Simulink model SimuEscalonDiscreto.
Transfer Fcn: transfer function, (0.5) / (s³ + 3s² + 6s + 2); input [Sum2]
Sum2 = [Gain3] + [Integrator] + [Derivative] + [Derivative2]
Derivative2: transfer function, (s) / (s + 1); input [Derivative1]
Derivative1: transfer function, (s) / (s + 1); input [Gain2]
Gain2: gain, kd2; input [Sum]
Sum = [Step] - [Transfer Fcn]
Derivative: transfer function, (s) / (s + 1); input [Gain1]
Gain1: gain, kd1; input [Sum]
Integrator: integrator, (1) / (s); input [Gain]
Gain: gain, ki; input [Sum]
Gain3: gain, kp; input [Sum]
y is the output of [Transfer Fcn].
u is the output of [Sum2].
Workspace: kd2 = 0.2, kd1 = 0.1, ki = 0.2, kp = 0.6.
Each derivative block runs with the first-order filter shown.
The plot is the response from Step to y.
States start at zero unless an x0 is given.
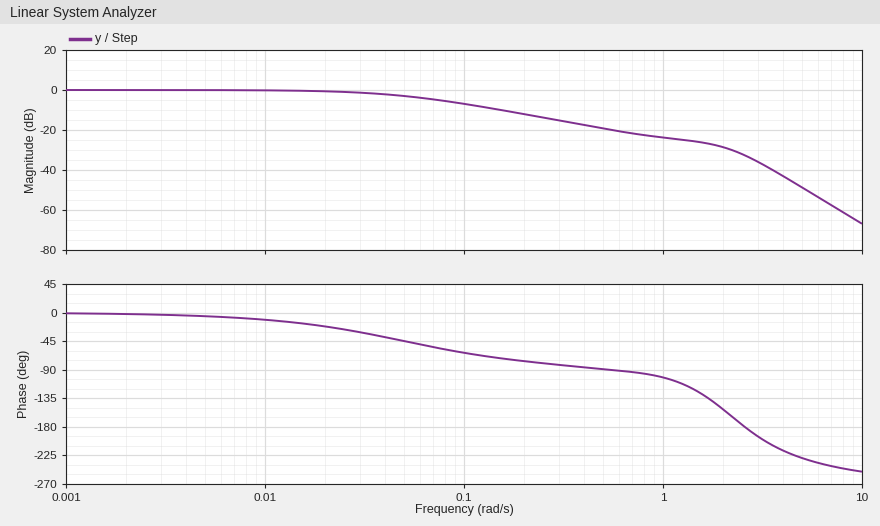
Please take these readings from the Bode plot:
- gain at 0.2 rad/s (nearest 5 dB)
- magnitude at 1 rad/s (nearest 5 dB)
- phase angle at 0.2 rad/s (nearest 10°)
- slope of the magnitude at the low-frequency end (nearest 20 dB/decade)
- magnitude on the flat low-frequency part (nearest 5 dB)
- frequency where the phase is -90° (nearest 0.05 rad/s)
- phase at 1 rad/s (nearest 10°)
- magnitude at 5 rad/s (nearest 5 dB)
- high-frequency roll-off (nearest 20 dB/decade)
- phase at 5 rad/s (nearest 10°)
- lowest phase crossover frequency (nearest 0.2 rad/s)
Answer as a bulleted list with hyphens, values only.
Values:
- -10 dB
- -25 dB
- -80°
- 0 dB/decade
- 0 dB
- 0.55 rad/s
- -100°
- -50 dB
- -60 dB/decade
- -230°
- 2.6 rad/s
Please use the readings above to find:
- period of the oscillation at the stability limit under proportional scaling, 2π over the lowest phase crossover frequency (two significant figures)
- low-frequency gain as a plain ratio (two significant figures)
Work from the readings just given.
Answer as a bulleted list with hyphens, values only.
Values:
- 2.4 s
- 1.0
